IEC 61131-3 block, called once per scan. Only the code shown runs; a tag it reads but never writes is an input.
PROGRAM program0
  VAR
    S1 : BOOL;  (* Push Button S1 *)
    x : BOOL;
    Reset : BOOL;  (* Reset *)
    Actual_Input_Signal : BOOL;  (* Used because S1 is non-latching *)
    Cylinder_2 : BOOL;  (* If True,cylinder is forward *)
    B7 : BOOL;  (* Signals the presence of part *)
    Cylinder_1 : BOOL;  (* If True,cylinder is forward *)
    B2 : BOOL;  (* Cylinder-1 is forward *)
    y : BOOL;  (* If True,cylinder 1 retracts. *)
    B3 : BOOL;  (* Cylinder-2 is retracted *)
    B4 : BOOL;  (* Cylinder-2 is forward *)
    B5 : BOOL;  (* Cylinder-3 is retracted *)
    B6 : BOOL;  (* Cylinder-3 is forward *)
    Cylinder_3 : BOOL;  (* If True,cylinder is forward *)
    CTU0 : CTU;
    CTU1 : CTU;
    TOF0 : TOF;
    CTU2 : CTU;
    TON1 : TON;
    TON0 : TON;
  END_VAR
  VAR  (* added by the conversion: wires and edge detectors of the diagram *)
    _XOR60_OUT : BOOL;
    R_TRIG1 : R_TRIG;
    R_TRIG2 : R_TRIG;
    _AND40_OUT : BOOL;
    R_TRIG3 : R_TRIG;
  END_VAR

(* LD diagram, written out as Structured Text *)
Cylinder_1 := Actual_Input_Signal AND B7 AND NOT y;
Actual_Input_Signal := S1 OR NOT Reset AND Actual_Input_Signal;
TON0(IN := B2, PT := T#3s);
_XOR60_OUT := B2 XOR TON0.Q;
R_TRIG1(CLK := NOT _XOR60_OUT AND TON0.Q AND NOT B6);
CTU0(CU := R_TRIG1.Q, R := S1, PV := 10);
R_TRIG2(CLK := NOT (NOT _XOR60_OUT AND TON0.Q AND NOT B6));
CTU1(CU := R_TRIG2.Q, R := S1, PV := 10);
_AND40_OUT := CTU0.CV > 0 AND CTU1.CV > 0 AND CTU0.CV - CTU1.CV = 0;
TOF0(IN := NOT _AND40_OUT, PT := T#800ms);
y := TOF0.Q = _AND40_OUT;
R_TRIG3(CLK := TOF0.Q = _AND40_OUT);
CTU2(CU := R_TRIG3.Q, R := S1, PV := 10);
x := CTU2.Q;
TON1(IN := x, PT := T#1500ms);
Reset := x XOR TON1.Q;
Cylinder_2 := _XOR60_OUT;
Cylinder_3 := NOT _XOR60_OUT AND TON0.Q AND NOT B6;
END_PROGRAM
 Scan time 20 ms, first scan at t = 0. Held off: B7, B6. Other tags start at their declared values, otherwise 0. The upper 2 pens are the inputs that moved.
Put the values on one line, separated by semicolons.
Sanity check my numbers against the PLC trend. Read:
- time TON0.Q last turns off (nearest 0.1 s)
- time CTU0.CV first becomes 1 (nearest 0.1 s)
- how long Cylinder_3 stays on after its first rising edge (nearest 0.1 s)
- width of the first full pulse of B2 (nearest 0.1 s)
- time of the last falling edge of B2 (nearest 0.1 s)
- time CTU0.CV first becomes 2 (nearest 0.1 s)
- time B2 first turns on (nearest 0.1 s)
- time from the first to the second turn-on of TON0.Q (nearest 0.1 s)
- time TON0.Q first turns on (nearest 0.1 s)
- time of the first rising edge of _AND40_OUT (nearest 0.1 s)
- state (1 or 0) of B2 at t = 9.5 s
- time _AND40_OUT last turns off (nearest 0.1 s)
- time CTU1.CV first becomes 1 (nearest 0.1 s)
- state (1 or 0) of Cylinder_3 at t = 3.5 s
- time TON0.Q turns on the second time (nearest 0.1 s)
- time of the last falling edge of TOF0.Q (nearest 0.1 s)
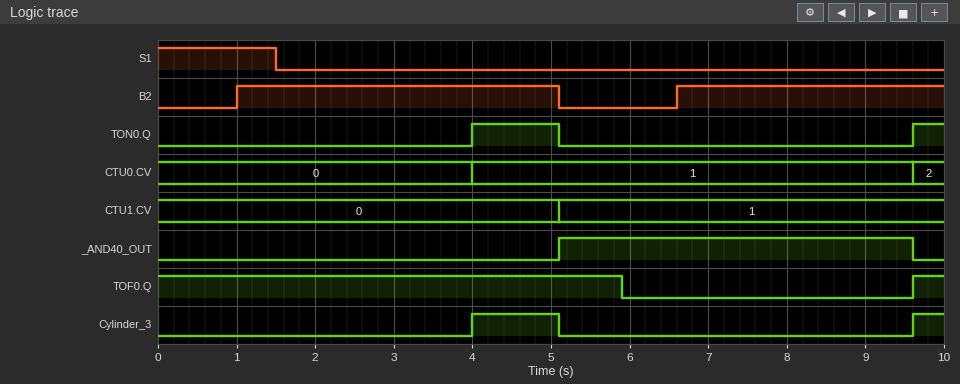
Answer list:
5.1 s; 4.0 s; 1.1 s; 4.1 s; 5.1 s; 9.6 s; 1.0 s; 5.6 s; 4.0 s; 5.1 s; 1; 9.6 s; 5.1 s; 0; 9.6 s; 5.9 s
